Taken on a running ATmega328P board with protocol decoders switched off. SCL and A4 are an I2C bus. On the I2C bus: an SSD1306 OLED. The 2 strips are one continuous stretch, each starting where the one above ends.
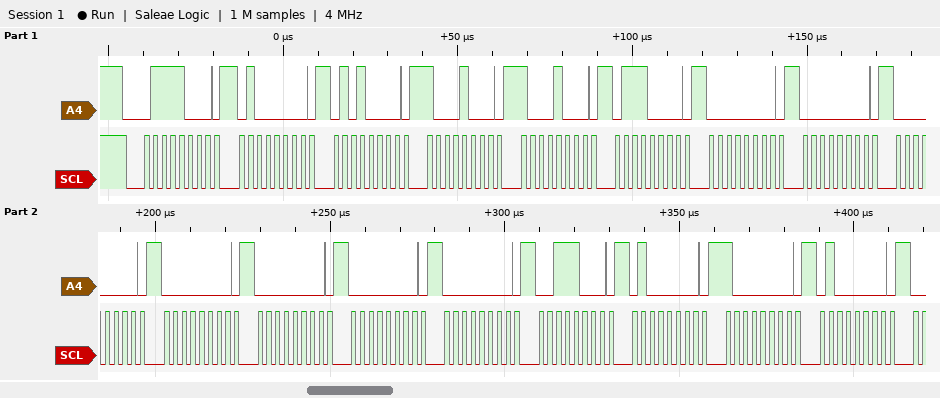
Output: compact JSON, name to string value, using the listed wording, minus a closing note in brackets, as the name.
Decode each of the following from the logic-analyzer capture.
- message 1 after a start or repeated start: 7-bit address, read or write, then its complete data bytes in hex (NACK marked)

{"message 1 after a start or repeated start: 7-bit address, read or write, then its complete data bytes in hex": "0x3C write: 40 50 88 88 70 00 00 00 00 00 00 00 38 40 80 40"}
